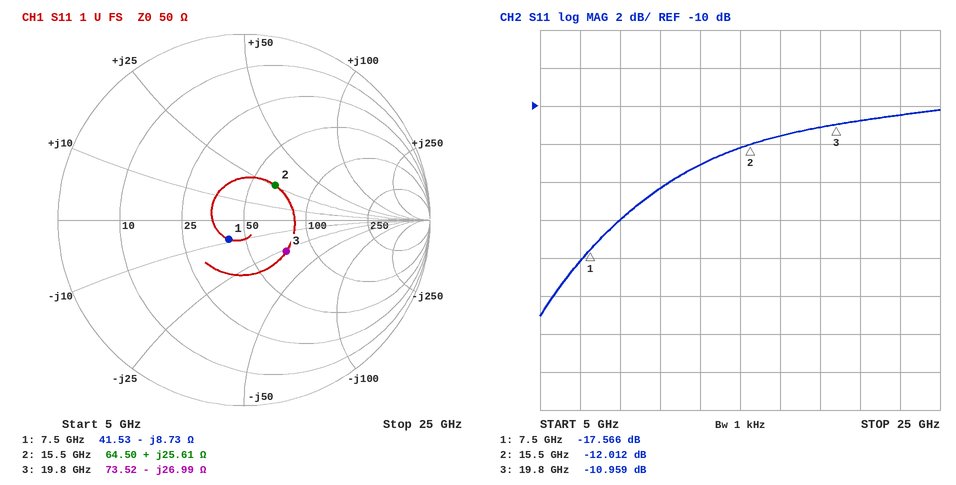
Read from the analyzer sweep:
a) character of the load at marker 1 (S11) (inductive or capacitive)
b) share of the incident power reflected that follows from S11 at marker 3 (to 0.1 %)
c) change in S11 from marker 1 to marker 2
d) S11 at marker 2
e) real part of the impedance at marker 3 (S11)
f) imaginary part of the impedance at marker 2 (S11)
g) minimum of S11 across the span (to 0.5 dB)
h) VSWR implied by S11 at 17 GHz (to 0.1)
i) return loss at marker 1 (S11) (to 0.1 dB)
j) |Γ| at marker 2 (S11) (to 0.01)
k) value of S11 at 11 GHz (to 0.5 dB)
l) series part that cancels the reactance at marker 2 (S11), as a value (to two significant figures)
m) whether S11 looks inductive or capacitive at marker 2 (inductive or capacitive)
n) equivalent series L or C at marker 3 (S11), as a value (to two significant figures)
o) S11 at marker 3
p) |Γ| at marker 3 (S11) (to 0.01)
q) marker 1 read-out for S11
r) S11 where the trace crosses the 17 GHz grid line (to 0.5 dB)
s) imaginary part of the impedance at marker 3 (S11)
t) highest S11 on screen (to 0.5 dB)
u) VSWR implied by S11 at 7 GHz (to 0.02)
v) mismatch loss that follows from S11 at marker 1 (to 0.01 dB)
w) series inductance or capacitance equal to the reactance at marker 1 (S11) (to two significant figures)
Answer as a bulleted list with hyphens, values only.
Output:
- capacitive
- 8.0 %
- 5.554 dB
- -12.012 dB
- 73.52 Ω
- +25.61 Ω
- -21.0 dB
- 1.7
- 17.6 dB
- 0.25
- -14.5 dB
- 400 fF
- inductive
- 300 fF
- -10.959 dB
- 0.28
- -17.566 dB
- -11.5 dB
- -26.99 Ω
- -10.0 dB
- 1.28
- 0.08 dB
- 2.4 pF
